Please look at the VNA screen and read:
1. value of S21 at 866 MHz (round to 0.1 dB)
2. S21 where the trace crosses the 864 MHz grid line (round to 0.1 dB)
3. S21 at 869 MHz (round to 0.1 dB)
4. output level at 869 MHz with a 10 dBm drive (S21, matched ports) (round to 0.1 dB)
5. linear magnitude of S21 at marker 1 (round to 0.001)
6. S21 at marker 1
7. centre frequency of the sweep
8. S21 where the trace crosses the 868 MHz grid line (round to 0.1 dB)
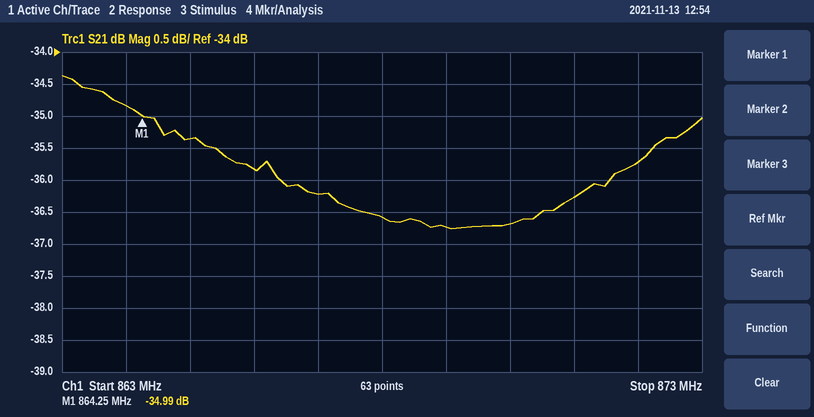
-35.8 dB
-34.8 dB
-36.7 dB
-26.7 dBm
0.018
-34.99 dB
868 MHz
-36.6 dB
